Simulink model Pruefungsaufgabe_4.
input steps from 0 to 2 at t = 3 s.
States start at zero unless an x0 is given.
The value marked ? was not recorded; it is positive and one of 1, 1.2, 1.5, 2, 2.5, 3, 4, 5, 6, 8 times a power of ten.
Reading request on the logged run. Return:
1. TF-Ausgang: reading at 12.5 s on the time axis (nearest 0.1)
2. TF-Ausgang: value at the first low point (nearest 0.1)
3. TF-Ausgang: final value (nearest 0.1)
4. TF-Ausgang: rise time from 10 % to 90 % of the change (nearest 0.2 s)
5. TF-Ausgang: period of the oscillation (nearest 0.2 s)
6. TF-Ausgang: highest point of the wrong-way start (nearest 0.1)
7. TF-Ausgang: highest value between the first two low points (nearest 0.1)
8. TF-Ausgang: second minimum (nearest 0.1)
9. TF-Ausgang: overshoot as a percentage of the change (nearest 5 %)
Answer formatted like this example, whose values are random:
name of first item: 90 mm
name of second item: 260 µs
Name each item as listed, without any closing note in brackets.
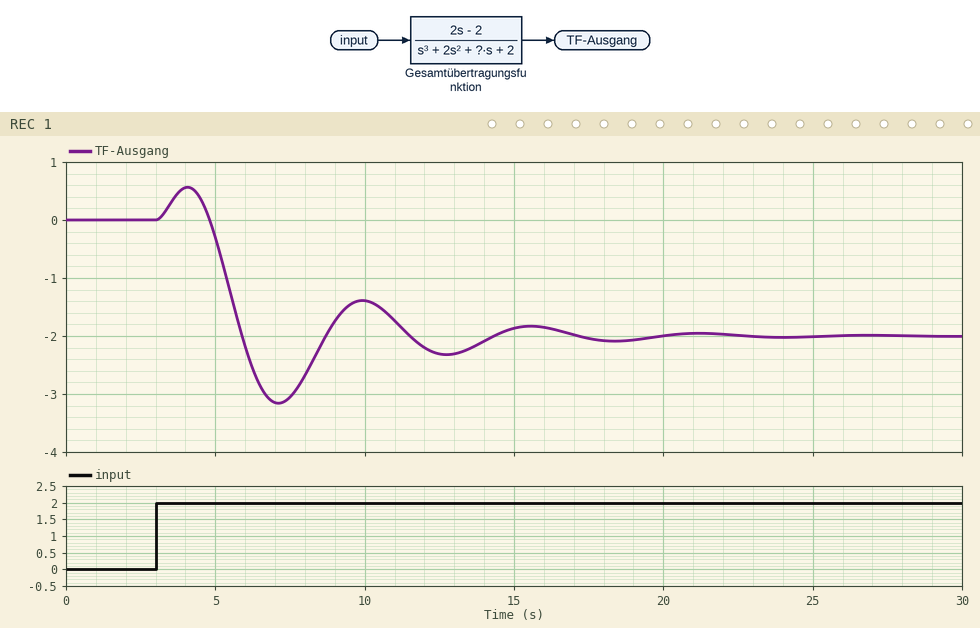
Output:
TF-Ausgang: reading at 12.5 s on the time axis: -2.3
TF-Ausgang: value at the first low point: -3.2
TF-Ausgang: final value: -2.0
TF-Ausgang: rise time from 10 % to 90 % of the change: 0.8 s
TF-Ausgang: period of the oscillation: 5.6 s
TF-Ausgang: highest point of the wrong-way start: 0.6
TF-Ausgang: highest value between the first two low points: -1.4
TF-Ausgang: second minimum: -2.3
TF-Ausgang: overshoot as a percentage of the change: 60 %
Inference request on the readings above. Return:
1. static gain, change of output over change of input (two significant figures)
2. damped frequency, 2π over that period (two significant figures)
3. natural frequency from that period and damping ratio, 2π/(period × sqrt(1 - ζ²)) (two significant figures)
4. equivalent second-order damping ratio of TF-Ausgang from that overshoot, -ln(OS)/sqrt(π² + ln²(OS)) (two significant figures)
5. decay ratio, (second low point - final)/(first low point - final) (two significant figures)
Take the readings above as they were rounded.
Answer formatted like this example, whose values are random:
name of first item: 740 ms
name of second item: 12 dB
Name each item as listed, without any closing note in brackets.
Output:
static gain, change of output over change of input: -1.0
damped frequency, 2π over that period: 1.1 rad/s
natural frequency from that period and damping ratio, 2π/(period × sqrt(1 - ζ²)): 1.1 rad/s
equivalent second-order damping ratio of TF-Ausgang from that overshoot, -ln(OS)/sqrt(π² + ln²(OS)): 0.16
decay ratio, (second low point - final)/(first low point - final): 0.25
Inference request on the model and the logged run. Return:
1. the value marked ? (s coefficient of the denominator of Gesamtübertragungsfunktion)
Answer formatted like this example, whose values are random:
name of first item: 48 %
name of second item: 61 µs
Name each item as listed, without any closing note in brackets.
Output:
the value marked ?: 2
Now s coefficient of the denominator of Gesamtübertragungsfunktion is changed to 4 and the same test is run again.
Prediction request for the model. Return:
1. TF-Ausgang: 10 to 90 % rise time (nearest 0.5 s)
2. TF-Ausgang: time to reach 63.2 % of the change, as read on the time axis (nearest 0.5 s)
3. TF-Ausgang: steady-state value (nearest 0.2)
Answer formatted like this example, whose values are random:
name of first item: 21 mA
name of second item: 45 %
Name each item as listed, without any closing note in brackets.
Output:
TF-Ausgang: 10 to 90 % rise time: 2.0 s
TF-Ausgang: time to reach 63.2 % of the change, as read on the time axis: 5.5 s
TF-Ausgang: steady-state value: -2.0
